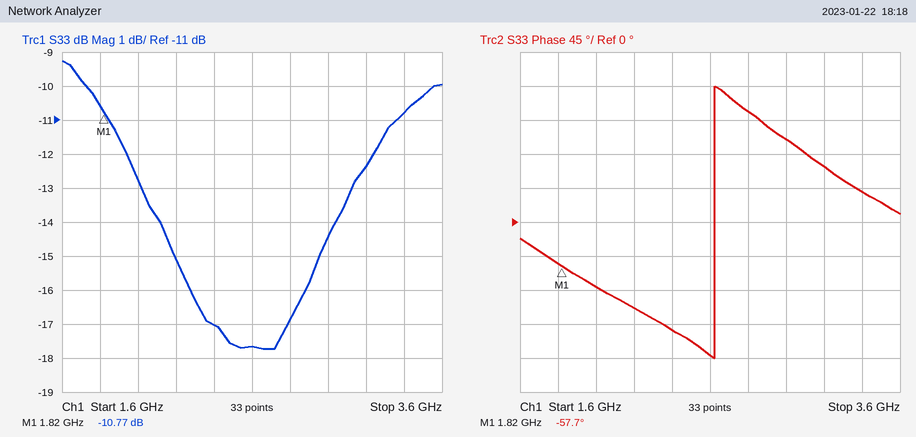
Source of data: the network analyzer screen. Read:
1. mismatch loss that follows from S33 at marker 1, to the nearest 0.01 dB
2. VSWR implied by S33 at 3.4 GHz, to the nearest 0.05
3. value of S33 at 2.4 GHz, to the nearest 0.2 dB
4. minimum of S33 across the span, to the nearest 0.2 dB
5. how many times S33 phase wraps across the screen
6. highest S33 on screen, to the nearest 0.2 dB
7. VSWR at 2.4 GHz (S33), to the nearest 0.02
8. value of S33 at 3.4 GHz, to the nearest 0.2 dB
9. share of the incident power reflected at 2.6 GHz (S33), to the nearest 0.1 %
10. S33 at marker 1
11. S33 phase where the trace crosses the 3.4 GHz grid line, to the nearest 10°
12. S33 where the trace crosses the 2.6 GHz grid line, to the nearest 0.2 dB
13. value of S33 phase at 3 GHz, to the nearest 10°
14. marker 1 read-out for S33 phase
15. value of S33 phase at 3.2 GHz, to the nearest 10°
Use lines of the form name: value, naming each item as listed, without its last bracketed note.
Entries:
mismatch loss that follows from S33 at marker 1, to the nearest 0.01 dB: 0.38 dB
VSWR implied by S33 at 3.4 GHz, to the nearest 0.05: 1.80
value of S33 at 2.4 GHz, to the nearest 0.2 dB: -17.0 dB
minimum of S33 across the span, to the nearest 0.2 dB: -17.8 dB
how many times S33 phase wraps across the screen: 1
highest S33 on screen, to the nearest 0.2 dB: -9.2 dB
VSWR at 2.4 GHz (S33), to the nearest 0.02: 1.32
value of S33 at 3.4 GHz, to the nearest 0.2 dB: -10.8 dB
share of the incident power reflected at 2.6 GHz (S33), to the nearest 0.1 %: 1.7 %
S33 at marker 1: -10.77 dB
S33 phase where the trace crosses the 3.4 GHz grid line, to the nearest 10°: 40°
S33 where the trace crosses the 2.6 GHz grid line, to the nearest 0.2 dB: -17.6 dB
value of S33 phase at 3 GHz, to the nearest 10°: 110°
marker 1 read-out for S33 phase: -57.7°
value of S33 phase at 3.2 GHz, to the nearest 10°: 70°
